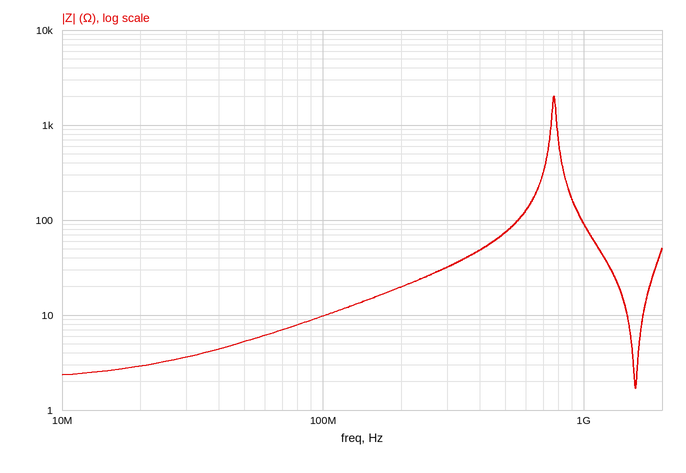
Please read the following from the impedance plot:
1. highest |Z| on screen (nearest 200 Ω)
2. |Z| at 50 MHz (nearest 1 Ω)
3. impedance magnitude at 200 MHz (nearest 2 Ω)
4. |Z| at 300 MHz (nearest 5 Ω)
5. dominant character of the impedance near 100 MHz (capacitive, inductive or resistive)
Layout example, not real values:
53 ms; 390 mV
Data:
2.0 kΩ; 5 Ω; 20 Ω; 30 Ω; inductive
